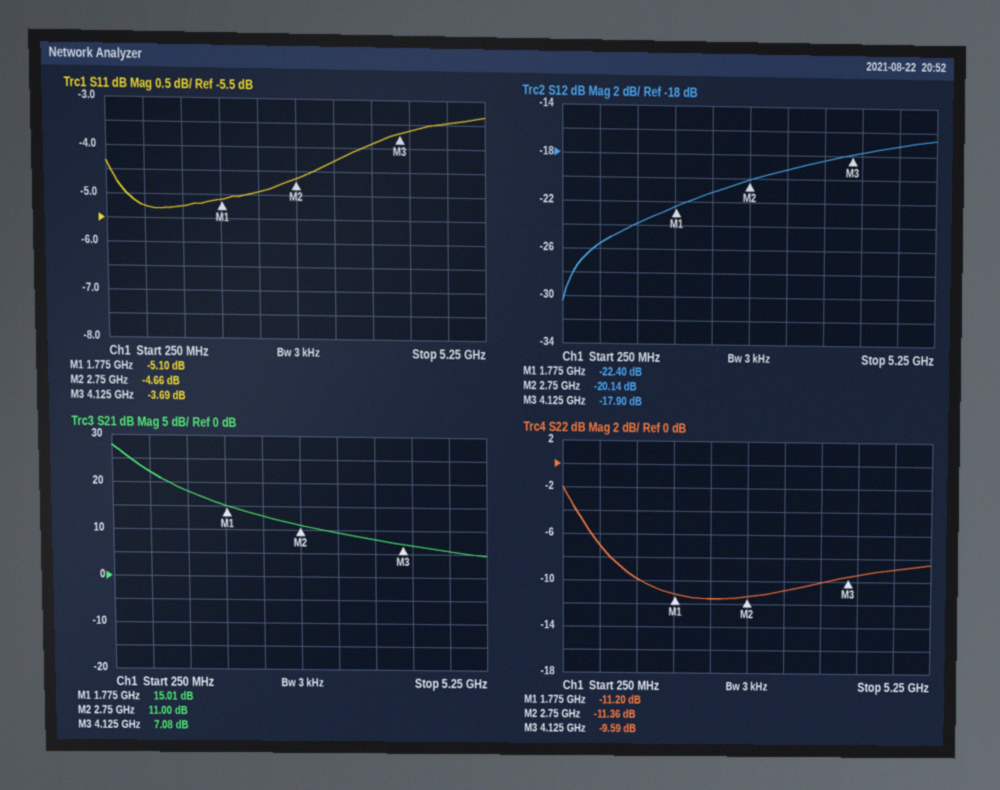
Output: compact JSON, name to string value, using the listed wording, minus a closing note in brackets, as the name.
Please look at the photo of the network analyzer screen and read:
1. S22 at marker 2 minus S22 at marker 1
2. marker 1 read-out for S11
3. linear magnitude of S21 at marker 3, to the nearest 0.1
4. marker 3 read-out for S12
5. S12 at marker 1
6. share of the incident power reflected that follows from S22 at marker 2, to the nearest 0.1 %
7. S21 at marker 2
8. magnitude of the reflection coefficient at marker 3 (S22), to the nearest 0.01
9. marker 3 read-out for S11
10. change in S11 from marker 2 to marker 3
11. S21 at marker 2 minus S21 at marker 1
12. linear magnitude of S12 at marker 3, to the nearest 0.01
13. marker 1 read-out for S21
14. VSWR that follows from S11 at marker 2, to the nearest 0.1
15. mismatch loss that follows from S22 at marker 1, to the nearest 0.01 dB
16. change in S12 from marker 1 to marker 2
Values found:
{"S22 at marker 2 minus S22 at marker 1": "-0.16 dB", "marker 1 read-out for S11": "-5.10 dB", "linear magnitude of S21 at marker 3, to the nearest 0.1": "2.3", "marker 3 read-out for S12": "-17.90 dB", "S12 at marker 1": "-22.40 dB", "share of the incident power reflected that follows from S22 at marker 2, to the nearest 0.1 %": "7.3 %", "S21 at marker 2": "11.00 dB", "magnitude of the reflection coefficient at marker 3 (S22), to the nearest 0.01": "0.33", "marker 3 read-out for S11": "-3.69 dB", "change in S11 from marker 2 to marker 3": "0.97 dB", "S21 at marker 2 minus S21 at marker 1": "-4.01 dB", "linear magnitude of S12 at marker 3, to the nearest 0.01": "0.13", "marker 1 read-out for S21": "15.01 dB", "VSWR that follows from S11 at marker 2, to the nearest 0.1": "3.8", "mismatch loss that follows from S22 at marker 1, to the nearest 0.01 dB": "0.34 dB", "change in S12 from marker 1 to marker 2": "2.26 dB"}
